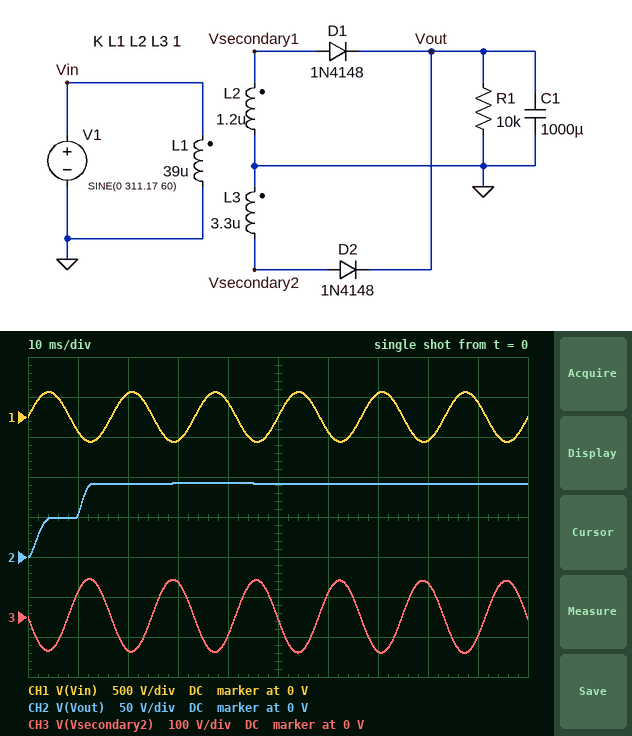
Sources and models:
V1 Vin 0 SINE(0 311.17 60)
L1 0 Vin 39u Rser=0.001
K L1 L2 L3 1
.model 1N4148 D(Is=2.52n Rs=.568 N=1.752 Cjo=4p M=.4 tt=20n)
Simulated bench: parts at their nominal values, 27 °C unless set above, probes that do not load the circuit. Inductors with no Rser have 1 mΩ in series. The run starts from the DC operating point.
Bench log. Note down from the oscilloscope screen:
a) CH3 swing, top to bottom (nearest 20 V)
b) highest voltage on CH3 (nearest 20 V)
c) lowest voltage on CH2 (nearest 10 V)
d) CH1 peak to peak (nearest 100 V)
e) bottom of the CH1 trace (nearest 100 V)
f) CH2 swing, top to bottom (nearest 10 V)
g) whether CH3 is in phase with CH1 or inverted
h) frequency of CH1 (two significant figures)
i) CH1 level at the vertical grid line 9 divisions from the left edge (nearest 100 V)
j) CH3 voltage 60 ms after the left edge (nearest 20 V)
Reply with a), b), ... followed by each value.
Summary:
a) 180 V
b) 100 V
c) 0 V
d) 600 V
e) -300 V
f) 90 V
g) inverted
h) 60 Hz
i) 200 V
j) 60 V
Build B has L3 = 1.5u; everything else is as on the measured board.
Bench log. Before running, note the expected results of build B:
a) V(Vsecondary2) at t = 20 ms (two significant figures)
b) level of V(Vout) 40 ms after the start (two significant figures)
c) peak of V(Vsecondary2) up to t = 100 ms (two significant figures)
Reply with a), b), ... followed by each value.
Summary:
a) -57 V
b) 62 V
c) 64 V
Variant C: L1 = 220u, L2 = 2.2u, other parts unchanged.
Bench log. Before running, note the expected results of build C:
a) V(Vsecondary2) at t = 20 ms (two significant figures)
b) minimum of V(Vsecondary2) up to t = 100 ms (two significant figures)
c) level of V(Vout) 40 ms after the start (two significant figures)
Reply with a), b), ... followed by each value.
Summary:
a) -36 V
b) -38 V
c) 37 V
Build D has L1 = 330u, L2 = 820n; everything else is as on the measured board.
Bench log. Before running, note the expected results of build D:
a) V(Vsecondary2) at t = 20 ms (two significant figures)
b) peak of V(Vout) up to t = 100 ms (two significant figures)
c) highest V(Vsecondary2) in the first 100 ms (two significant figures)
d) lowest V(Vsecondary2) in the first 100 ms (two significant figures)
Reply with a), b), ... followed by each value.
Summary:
a) -29 V
b) 30 V
c) 31 V
d) -31 V
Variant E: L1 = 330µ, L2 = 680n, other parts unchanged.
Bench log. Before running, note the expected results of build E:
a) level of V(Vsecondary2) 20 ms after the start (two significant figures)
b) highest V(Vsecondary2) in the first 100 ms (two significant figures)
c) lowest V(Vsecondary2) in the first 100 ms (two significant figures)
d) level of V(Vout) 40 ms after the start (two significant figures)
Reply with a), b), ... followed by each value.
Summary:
a) -29 V
b) 31 V
c) -31 V
d) 30 V
